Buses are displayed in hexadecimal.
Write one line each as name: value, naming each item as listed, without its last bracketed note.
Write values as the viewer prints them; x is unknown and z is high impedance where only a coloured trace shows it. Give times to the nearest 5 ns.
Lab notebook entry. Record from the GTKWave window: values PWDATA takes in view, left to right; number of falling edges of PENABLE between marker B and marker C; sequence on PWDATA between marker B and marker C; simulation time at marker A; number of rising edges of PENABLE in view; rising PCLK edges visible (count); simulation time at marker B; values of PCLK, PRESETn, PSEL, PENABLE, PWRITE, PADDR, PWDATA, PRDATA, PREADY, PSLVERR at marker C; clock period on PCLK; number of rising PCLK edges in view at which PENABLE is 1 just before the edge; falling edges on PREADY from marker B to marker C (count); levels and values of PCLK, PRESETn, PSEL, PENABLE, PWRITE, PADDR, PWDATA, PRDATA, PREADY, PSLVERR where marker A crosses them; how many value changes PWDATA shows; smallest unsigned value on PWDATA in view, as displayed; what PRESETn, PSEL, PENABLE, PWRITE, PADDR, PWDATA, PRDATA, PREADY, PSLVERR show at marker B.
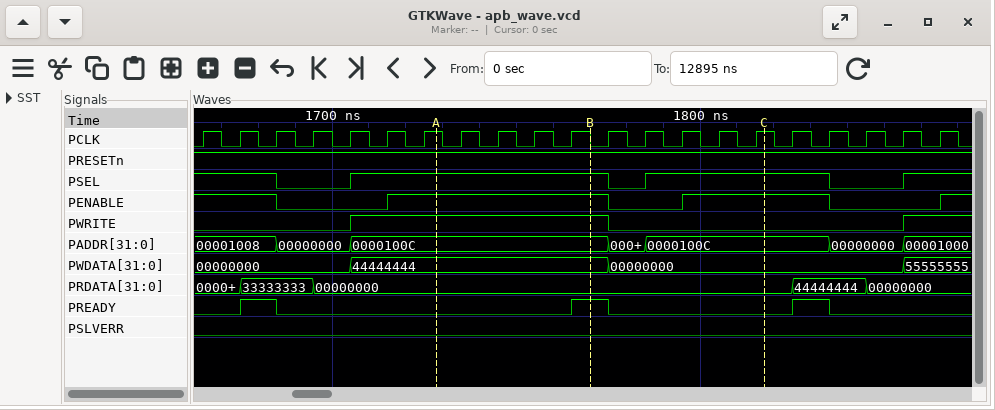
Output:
values PWDATA takes in view, left to right: 00000000, 44444444, 00000000, 55555555
number of falling edges of PENABLE between marker B and marker C: 1
sequence on PWDATA between marker B and marker C: 44444444, 00000000
simulation time at marker A: 1730 ns
number of rising edges of PENABLE in view: 3
rising PCLK edges visible: 21
simulation time at marker B: 1770 ns
values of PCLK, PRESETn, PSEL, PENABLE, PWRITE, PADDR, PWDATA, PRDATA, PREADY, PSLVERR at marker C: PCLK=1, PRESETn=1, PSEL=1, PENABLE=1, PWRITE=0, PADDR=0000100C, PWDATA=00000000, PRDATA=00000000, PREADY=0, PSLVERR=0
clock period on PCLK: 10 ns
number of rising PCLK edges in view at which PENABLE is 1 just before the edge: 13
falling edges on PREADY from marker B to marker C: 1
levels and values of PCLK, PRESETn, PSEL, PENABLE, PWRITE, PADDR, PWDATA, PRDATA, PREADY, PSLVERR where marker A crosses them: PCLK=1, PRESETn=1, PSEL=1, PENABLE=1, PWRITE=1, PADDR=0000100C, PWDATA=44444444, PRDATA=00000000, PREADY=0, PSLVERR=0
how many value changes PWDATA shows: 3
smallest unsigned value on PWDATA in view, as displayed: 00000000
what PRESETn, PSEL, PENABLE, PWRITE, PADDR, PWDATA, PRDATA, PREADY, PSLVERR show at marker B: PRESETn=1, PSEL=1, PENABLE=1, PWRITE=1, PADDR=0000100C, PWDATA=44444444, PRDATA=00000000, PREADY=1, PSLVERR=0
